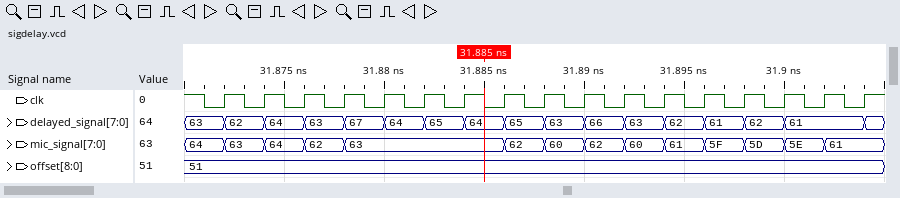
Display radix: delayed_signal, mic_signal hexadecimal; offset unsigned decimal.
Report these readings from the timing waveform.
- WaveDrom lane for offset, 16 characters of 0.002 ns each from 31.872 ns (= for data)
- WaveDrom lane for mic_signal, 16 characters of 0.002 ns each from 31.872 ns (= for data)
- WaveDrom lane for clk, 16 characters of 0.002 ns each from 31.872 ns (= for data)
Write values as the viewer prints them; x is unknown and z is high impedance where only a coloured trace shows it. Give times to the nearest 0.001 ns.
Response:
{name: 'offset', wave: '=...............', data: '51'}
{name: 'mic_signal', wave: '====...=========', data: '63 64 62 63 62 60 62 60 61 5F 5D 5E 61'}
{name: 'clk', wave: 'p...............'}
